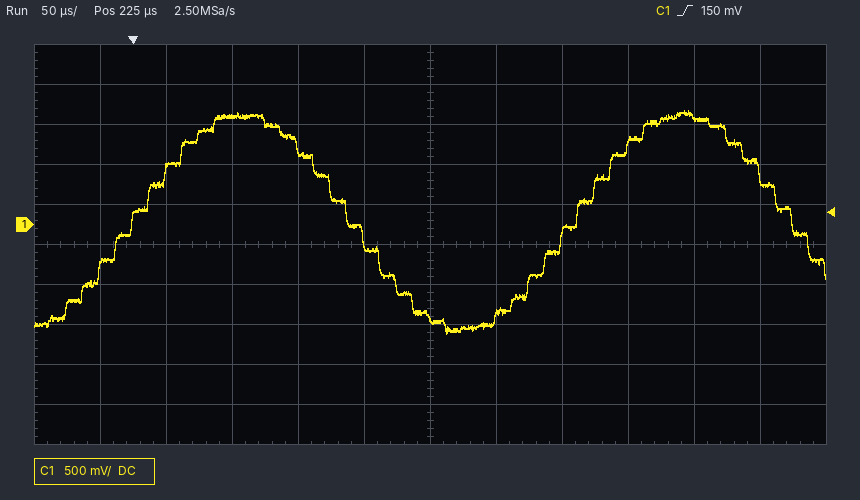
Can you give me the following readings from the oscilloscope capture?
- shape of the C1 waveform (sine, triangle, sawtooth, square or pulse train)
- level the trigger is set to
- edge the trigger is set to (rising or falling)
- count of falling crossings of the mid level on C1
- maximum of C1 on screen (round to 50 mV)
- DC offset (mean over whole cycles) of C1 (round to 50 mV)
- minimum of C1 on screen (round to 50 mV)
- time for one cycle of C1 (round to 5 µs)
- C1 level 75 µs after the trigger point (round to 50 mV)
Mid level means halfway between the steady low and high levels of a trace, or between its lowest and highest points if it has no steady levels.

sine
150 mV
rising
2
1.40 V
50 mV
-1.35 V
335 µs
1.35 V
